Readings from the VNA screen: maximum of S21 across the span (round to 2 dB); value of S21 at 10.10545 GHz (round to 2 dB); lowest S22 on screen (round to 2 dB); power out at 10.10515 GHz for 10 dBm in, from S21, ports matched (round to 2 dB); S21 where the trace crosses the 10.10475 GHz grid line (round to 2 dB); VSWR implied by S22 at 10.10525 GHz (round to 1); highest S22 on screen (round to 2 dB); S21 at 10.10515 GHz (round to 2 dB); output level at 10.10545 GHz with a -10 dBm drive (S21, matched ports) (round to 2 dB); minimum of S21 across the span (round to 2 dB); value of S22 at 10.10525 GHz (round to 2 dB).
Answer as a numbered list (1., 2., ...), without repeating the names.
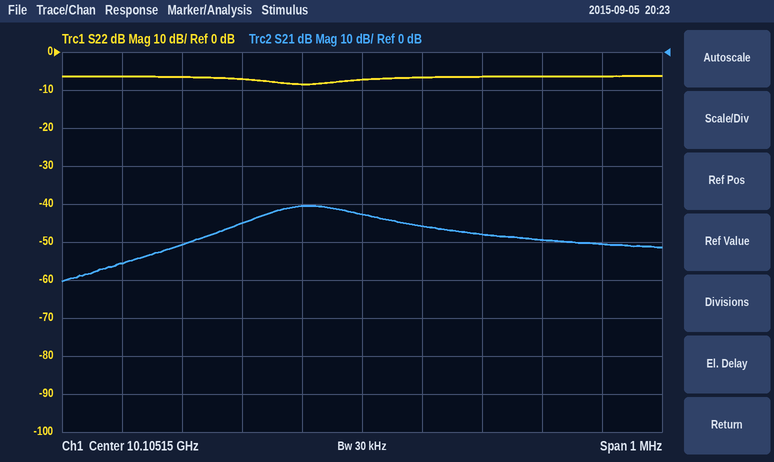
1. -40 dB
2. -50 dB
3. -8 dB
4. -32 dBm
5. -56 dB
6. 3
7. -6 dB
8. -42 dB
9. -60 dBm
10. -60 dB
11. -6 dB
